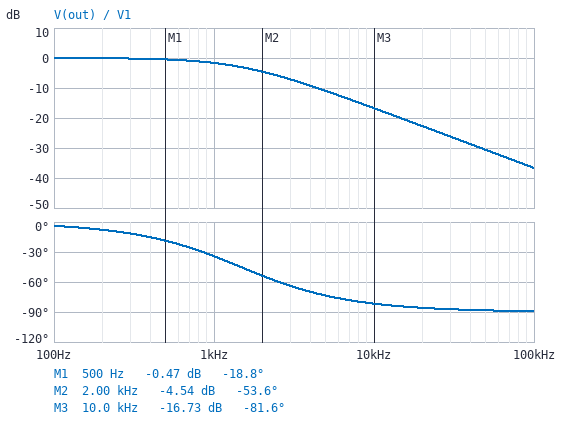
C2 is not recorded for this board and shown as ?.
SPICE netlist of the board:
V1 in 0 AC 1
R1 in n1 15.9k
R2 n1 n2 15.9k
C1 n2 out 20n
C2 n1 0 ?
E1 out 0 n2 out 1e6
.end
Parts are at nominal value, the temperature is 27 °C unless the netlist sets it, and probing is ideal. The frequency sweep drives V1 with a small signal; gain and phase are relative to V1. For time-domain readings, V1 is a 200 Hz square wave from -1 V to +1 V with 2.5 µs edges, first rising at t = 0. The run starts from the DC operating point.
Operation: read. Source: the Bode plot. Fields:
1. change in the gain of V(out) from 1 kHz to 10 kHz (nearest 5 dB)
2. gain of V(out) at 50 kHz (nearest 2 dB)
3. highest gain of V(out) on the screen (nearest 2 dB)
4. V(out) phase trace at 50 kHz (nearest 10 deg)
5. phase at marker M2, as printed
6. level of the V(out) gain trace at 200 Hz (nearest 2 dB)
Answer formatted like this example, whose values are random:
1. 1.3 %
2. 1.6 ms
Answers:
1. -15 dB
2. -30 dB
3. 0 dB
4. -90 deg
5. -53.6 deg
6. 0 dB
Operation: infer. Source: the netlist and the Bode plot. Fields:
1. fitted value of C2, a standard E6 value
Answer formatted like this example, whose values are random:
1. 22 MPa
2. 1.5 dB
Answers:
1. 6.8 nF
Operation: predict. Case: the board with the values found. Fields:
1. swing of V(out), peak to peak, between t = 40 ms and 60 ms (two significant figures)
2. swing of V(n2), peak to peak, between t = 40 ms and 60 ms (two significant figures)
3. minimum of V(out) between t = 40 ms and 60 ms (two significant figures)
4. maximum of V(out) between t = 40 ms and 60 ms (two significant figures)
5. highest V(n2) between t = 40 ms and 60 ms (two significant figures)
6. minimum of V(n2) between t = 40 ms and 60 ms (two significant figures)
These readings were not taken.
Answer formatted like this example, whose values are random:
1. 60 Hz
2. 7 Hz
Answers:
1. 2.0 V
2. 2.0 V
3. -1.0 V
4. 1.0 V
5. 1.0 V
6. -1.0 V
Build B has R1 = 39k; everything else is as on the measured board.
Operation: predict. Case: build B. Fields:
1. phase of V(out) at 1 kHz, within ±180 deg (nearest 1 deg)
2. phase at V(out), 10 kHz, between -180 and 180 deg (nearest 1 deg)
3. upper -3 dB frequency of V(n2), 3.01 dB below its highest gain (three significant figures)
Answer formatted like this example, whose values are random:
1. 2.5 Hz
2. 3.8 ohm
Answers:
1. -59 deg
2. -87 deg
3. 600 Hz
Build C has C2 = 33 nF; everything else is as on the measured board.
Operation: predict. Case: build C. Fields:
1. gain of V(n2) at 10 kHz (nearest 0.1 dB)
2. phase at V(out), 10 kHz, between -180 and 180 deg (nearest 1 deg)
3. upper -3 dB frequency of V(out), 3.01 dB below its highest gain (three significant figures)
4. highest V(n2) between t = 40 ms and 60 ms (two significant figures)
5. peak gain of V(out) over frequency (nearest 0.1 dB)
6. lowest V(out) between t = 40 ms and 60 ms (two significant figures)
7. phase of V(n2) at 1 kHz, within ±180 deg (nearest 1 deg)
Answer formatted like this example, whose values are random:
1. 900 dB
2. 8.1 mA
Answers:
1. -30.4 dB
2. -88 deg
3. 303 Hz
4. 980 mV
5. 0 dB
6. -980 mV
7. -73 deg
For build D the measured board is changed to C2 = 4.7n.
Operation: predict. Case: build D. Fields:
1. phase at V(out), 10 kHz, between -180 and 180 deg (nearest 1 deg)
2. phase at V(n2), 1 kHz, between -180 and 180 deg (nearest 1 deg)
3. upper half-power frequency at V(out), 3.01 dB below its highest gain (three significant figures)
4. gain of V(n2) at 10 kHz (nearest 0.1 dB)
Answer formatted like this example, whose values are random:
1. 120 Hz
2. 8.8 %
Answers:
1. -78 deg
2. -25 deg
3. 2.13 kHz
4. -13.6 dB
